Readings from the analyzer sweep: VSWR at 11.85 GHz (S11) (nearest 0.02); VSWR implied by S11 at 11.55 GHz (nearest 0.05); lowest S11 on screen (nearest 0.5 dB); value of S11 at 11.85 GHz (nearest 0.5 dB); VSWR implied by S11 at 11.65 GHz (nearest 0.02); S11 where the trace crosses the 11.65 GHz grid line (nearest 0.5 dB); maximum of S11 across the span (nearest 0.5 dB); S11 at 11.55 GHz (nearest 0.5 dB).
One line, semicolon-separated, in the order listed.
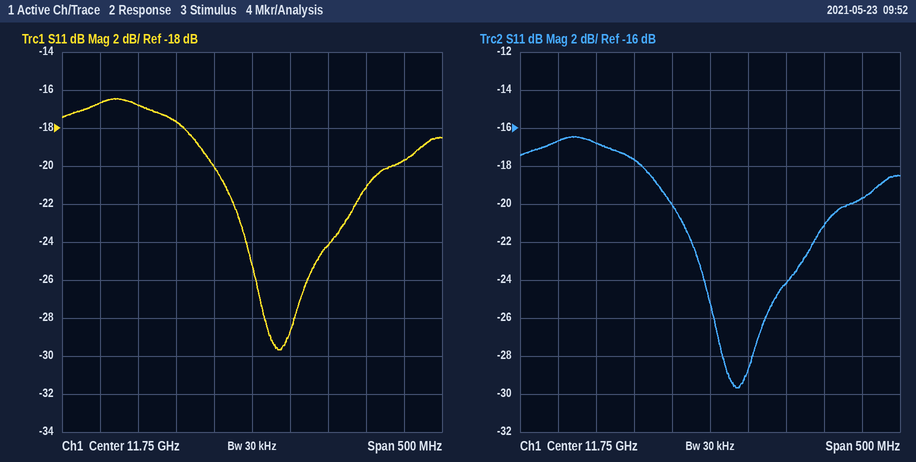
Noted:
1.14; 1.35; -29.5 dB; -24.0 dB; 1.30; -17.5 dB; -16.5 dB; -16.5 dB
